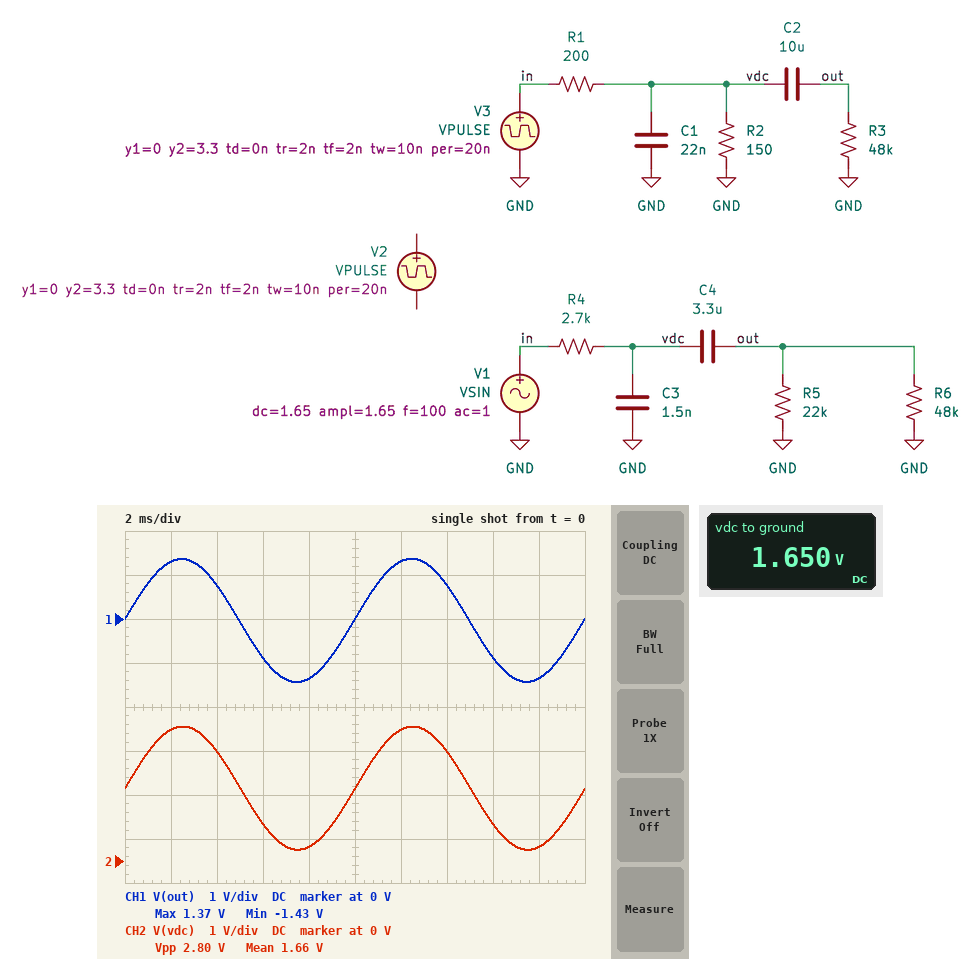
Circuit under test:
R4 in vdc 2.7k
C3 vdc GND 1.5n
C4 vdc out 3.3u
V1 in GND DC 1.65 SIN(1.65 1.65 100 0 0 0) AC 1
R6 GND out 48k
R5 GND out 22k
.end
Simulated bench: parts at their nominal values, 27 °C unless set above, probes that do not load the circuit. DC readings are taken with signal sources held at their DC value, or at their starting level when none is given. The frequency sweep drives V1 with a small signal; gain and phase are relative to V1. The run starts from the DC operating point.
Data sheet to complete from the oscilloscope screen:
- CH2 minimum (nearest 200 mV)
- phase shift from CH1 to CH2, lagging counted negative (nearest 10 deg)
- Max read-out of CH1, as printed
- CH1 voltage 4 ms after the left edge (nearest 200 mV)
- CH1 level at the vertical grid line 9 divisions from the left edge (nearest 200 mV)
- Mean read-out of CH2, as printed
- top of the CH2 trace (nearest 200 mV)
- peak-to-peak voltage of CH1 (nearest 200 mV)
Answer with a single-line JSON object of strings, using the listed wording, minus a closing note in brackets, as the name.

{"CH2 minimum": "200 mV", "phase shift from CH1 to CH2, lagging counted negative": "0 deg", "Max read-out of CH1, as printed": "1.37 V", "CH1 voltage 4 ms after the left edge": "800 mV", "CH1 level at the vertical grid line 9 divisions from the left edge": "-1.4 V", "Mean read-out of CH2, as printed": "1.66 V", "top of the CH2 trace": "3.0 V", "peak-to-peak voltage of CH1": "2.8 V"}
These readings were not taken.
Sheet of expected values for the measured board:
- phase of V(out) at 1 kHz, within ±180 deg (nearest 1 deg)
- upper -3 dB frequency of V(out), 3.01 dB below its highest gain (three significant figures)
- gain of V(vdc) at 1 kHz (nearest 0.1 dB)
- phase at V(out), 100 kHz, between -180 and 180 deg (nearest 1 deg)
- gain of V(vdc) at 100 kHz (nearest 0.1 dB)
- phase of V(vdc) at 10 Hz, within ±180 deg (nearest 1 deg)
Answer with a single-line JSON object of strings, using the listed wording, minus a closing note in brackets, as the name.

{"phase of V(out) at 1 kHz, within ±180 deg": "-1 deg", "upper -3 dB frequency of V(out), 3.01 dB below its highest gain": "46.3 kHz", "gain of V(vdc) at 1 kHz": "-1.4 dB", "phase at V(out), 100 kHz, between -180 and 180 deg": "-65 deg", "gain of V(vdc) at 100 kHz": "-9.0 dB", "phase of V(vdc) at 10 Hz, within ±180 deg": "-3 deg"}
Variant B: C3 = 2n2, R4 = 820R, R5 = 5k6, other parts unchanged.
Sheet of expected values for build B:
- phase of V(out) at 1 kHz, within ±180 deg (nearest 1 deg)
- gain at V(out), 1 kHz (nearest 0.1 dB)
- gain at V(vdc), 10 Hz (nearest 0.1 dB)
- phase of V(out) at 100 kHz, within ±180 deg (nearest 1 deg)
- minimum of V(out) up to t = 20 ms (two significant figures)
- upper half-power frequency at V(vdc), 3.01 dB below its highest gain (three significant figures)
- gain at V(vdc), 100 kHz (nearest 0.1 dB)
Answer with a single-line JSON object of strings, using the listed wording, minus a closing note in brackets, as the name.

{"phase of V(out) at 1 kHz, within ±180 deg": "0 deg", "gain at V(out), 1 kHz": "-1.3 dB", "gain at V(vdc), 10 Hz": "-0.7 dB", "phase of V(out) at 100 kHz, within ±180 deg": "-44 deg", "minimum of V(out) up to t = 20 ms": "-1.5 V", "upper half-power frequency at V(vdc), 3.01 dB below its highest gain": "70.9 kHz", "gain at V(vdc), 100 kHz": "-4.2 dB"}
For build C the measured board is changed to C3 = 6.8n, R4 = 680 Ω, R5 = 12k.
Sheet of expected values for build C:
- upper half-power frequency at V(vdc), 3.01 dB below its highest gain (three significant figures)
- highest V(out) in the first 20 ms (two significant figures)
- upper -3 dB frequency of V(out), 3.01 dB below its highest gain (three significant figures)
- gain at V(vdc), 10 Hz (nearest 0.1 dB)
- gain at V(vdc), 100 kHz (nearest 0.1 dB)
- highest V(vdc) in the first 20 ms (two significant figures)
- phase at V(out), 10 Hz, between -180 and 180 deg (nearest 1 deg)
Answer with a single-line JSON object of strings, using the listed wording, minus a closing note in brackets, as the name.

{"upper half-power frequency at V(vdc), 3.01 dB below its highest gain": "31.8 kHz", "highest V(out) in the first 20 ms": "1.5 V", "upper -3 dB frequency of V(out), 3.01 dB below its highest gain": "36.9 kHz", "gain at V(vdc), 10 Hz": "-0.5 dB", "gain at V(vdc), 100 kHz": "-9.8 dB", "highest V(vdc) in the first 20 ms": "3.2 V", "phase at V(out), 10 Hz, between -180 and 180 deg": "25 deg"}
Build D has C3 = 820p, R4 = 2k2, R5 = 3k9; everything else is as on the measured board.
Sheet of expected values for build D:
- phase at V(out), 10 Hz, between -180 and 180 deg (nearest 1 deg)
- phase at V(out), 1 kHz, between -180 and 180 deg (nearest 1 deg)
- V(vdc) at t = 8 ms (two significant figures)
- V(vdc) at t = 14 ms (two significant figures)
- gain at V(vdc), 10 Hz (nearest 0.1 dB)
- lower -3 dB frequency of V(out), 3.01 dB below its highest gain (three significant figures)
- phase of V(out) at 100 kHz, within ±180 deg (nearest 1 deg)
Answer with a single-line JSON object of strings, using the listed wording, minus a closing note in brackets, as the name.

{"phase at V(out), 10 Hz, between -180 and 180 deg": "40 deg", "phase at V(out), 1 kHz, between -180 and 180 deg": "0 deg", "V(vdc) at t = 8 ms": "690 mV", "V(vdc) at t = 14 ms": "2.3 V", "gain at V(vdc), 10 Hz": "-2.0 dB", "lower -3 dB frequency of V(out), 3.01 dB below its highest gain": "8.30 Hz", "phase of V(out) at 100 kHz, within ±180 deg": "-35 deg"}
